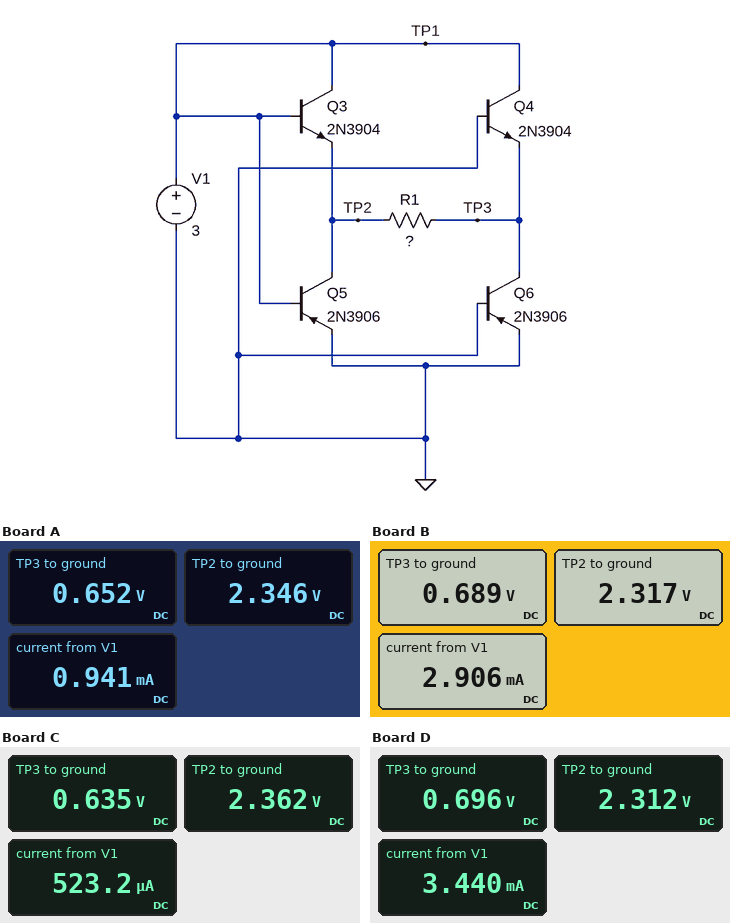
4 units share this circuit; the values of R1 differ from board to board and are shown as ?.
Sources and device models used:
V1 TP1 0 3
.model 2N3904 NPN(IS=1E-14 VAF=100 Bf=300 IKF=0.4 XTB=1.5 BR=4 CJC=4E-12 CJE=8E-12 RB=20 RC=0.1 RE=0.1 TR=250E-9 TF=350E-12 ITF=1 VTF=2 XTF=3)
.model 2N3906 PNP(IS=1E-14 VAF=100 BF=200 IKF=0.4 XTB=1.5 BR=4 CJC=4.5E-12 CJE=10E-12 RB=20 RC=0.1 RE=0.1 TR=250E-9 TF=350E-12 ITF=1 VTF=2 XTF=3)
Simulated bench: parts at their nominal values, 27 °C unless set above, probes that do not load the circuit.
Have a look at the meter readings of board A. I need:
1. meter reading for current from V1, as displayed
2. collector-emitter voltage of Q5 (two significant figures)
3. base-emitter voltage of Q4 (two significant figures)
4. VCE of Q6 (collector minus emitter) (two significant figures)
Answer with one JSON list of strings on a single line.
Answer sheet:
["0.941 mA", "2.3 V", "-650 mV", "650 mV"]
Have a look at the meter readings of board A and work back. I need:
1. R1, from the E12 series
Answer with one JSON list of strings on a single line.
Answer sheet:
["1.8 kΩ"]
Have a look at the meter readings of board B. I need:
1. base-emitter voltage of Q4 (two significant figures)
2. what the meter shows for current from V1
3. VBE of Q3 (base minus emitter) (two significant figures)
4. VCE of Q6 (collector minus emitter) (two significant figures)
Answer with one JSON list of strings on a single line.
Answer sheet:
["-690 mV", "2.906 mA", "680 mV", "690 mV"]
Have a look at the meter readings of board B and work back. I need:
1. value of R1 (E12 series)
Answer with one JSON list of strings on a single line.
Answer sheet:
["560 Ω"]
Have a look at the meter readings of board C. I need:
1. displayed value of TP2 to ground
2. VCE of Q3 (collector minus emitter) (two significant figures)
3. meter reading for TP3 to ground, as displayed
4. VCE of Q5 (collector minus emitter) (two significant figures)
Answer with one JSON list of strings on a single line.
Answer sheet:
["2.362 V", "640 mV", "0.635 V", "2.4 V"]
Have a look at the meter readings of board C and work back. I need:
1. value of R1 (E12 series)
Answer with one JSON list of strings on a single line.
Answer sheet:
["3.3 kΩ"]
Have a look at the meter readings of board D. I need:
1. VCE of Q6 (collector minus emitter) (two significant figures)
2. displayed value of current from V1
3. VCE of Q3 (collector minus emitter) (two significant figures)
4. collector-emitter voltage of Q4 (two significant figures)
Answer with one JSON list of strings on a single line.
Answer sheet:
["700 mV", "3.440 mA", "690 mV", "2.3 V"]
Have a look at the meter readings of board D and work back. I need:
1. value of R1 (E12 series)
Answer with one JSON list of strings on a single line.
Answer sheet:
["470 Ω"]
